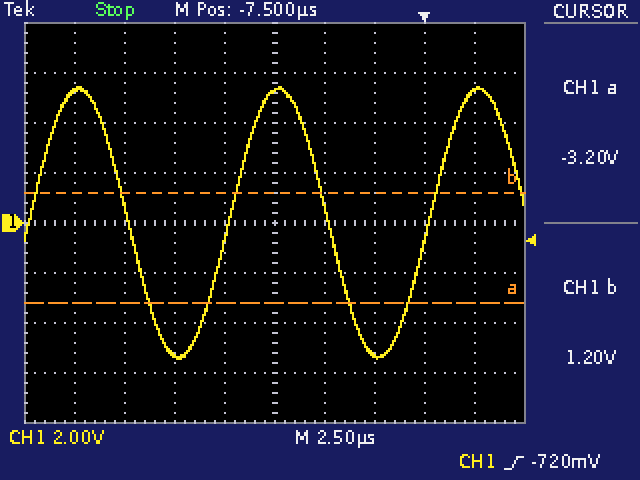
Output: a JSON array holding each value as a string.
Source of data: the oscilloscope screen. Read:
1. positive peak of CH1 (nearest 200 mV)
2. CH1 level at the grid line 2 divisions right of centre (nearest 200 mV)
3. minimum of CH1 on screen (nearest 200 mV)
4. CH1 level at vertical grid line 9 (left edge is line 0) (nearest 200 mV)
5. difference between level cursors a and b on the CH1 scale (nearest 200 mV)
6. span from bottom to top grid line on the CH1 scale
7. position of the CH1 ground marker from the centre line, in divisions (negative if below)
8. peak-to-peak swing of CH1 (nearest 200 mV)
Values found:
["5.4 V", "-5.2 V", "-5.4 V", "5.2 V", "4.4 V", "16 V", "0.0 div", "10.8 V"]
